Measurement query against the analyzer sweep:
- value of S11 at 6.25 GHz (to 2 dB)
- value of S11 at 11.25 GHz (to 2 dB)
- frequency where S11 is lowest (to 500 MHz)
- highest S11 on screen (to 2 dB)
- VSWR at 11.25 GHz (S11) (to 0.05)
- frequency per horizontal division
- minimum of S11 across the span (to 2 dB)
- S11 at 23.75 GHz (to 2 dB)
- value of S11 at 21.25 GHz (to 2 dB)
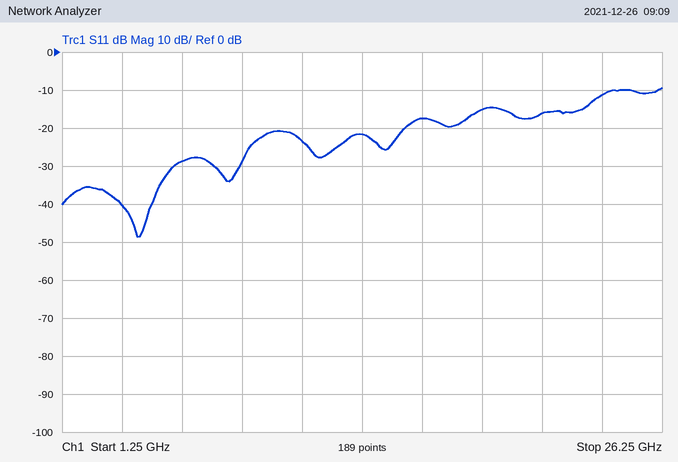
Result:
-28 dB
-24 dB
4.5 GHz
-10 dB
1.15
2.5 GHz
-48 dB
-12 dB
-16 dB
